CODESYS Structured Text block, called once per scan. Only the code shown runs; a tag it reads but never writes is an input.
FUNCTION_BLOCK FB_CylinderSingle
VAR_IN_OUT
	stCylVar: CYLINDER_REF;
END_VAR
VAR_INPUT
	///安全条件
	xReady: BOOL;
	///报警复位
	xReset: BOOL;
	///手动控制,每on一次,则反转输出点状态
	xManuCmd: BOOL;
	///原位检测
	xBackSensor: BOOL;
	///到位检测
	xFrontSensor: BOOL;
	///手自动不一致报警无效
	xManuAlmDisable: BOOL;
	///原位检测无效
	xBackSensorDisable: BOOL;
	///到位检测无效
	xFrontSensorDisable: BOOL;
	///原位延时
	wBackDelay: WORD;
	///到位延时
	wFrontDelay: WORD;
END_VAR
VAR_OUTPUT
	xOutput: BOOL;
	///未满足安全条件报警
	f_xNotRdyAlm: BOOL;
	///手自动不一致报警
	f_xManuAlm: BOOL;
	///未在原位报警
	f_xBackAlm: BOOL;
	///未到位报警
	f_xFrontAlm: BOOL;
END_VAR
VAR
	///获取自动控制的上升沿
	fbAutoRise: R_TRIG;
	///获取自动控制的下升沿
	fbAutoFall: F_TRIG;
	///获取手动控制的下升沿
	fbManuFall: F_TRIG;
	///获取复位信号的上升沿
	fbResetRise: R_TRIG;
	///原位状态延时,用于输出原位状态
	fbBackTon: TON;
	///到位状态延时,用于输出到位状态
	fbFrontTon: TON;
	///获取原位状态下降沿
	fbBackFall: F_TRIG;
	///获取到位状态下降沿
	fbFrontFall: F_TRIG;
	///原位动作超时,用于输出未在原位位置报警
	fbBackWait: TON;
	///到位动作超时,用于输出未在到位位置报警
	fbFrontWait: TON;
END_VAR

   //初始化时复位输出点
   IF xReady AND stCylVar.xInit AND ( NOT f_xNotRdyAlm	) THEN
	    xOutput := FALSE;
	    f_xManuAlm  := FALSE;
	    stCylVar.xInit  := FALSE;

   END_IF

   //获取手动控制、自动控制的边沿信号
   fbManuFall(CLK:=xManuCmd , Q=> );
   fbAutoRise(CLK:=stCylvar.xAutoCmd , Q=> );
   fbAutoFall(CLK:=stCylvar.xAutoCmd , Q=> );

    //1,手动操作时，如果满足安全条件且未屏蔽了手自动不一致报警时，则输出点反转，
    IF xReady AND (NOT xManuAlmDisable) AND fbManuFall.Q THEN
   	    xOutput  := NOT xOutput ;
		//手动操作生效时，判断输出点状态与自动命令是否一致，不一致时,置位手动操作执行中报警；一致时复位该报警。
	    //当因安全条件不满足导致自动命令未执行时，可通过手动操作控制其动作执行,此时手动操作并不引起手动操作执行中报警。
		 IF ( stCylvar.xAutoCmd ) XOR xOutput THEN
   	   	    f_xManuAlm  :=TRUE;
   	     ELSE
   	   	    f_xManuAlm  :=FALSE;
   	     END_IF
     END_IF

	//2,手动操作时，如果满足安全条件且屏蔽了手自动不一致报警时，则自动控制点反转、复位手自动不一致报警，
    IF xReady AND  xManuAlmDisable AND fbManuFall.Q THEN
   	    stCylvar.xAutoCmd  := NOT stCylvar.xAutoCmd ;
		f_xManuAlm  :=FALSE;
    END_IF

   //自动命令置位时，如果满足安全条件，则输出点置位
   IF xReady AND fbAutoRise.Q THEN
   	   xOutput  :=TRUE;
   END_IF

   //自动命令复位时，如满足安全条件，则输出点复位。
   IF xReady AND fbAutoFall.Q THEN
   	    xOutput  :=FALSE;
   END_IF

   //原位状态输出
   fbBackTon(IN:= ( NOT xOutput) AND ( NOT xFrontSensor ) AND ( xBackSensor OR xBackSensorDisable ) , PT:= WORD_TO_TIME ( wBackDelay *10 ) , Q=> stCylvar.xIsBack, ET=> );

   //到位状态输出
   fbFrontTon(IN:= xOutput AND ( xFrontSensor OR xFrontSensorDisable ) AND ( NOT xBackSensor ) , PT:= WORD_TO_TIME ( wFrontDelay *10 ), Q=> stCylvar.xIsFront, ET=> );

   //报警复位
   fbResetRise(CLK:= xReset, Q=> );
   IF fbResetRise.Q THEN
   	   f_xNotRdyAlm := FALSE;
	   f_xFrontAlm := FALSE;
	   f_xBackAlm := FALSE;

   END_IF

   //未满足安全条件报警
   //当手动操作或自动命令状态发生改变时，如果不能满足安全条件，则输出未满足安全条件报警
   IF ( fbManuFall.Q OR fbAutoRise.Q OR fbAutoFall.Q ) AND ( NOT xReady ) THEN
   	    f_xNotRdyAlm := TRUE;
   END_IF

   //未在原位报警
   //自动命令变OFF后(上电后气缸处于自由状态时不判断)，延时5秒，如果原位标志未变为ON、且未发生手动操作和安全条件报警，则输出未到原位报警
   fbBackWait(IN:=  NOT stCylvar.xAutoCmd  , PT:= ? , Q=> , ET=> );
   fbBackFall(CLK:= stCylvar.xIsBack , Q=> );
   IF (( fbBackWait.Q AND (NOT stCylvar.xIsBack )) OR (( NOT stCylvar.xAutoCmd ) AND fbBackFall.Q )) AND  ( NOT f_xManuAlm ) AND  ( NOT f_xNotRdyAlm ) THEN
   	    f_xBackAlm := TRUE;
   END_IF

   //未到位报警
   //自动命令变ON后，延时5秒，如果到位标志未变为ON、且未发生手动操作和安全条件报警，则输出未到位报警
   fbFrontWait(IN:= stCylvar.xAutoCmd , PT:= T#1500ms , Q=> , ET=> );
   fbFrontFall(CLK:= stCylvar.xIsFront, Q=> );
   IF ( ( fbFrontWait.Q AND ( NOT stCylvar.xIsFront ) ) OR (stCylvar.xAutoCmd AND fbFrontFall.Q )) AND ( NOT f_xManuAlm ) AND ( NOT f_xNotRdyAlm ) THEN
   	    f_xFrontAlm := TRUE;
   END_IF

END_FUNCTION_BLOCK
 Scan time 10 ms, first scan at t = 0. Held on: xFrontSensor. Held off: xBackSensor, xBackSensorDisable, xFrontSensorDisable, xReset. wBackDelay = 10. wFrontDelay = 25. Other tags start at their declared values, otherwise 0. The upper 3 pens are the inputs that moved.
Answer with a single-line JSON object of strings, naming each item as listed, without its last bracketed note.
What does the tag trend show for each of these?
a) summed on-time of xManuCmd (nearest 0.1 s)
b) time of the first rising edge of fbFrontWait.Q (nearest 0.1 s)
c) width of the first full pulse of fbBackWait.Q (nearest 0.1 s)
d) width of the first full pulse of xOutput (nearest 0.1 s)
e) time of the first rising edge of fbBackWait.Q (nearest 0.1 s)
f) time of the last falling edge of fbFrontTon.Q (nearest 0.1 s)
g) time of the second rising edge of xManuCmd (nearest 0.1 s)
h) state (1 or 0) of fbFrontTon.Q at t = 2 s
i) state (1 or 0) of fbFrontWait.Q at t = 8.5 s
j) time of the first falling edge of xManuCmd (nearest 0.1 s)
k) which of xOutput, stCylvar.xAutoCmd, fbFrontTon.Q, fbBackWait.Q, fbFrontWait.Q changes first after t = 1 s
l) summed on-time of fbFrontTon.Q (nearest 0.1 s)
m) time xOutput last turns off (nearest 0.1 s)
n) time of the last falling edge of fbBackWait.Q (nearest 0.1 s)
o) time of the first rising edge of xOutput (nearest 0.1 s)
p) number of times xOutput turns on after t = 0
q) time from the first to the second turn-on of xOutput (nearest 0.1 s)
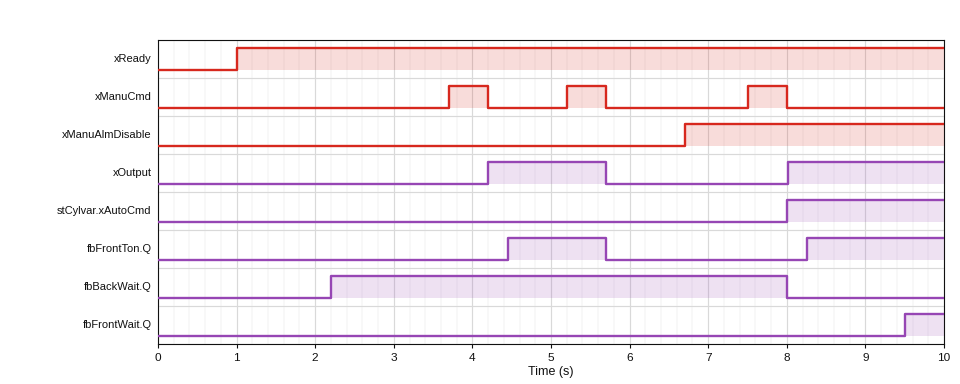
{"summed on-time of xManuCmd": "1.5 s", "time of the first rising edge of fbFrontWait.Q": "9.5 s", "width of the first full pulse of fbBackWait.Q": "5.8 s", "width of the first full pulse of xOutput": "1.5 s", "time of the first rising edge of fbBackWait.Q": "2.2 s", "time of the last falling edge of fbFrontTon.Q": "5.7 s", "time of the second rising edge of xManuCmd": "5.2 s", "state (1 or 0) of fbFrontTon.Q at t = 2 s": "0", "state (1 or 0) of fbFrontWait.Q at t = 8.5 s": "0", "time of the first falling edge of xManuCmd": "4.2 s", "which of xOutput, stCylvar.xAutoCmd, fbFrontTon.Q, fbBackWait.Q, fbFrontWait.Q changes first after t = 1 s": "fbBackWait.Q", "summed on-time of fbFrontTon.Q": "3.0 s", "time xOutput last turns off": "5.7 s", "time of the last falling edge of fbBackWait.Q": "8.0 s", "time of the first rising edge of xOutput": "4.2 s", "number of times xOutput turns on after t = 0": "2", "time from the first to the second turn-on of xOutput": "3.8 s"}
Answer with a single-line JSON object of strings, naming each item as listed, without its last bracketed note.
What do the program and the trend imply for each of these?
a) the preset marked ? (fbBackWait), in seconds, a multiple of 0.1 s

{"the preset marked ? (fbBackWait), in seconds, a multiple of 0.1 s": "2.2 s"}
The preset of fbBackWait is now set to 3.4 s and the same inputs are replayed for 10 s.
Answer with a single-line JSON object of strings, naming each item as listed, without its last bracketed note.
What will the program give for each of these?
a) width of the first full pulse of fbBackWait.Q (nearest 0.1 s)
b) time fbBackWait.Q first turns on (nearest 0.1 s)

{"width of the first full pulse of fbBackWait.Q": "4.6 s", "time fbBackWait.Q first turns on": "3.4 s"}
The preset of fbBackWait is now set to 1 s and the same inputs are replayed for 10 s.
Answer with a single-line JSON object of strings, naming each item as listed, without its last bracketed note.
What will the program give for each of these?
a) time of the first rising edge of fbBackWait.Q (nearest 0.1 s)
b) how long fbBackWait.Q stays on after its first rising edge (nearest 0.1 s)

{"time of the first rising edge of fbBackWait.Q": "1.0 s", "how long fbBackWait.Q stays on after its first rising edge": "7.0 s"}
